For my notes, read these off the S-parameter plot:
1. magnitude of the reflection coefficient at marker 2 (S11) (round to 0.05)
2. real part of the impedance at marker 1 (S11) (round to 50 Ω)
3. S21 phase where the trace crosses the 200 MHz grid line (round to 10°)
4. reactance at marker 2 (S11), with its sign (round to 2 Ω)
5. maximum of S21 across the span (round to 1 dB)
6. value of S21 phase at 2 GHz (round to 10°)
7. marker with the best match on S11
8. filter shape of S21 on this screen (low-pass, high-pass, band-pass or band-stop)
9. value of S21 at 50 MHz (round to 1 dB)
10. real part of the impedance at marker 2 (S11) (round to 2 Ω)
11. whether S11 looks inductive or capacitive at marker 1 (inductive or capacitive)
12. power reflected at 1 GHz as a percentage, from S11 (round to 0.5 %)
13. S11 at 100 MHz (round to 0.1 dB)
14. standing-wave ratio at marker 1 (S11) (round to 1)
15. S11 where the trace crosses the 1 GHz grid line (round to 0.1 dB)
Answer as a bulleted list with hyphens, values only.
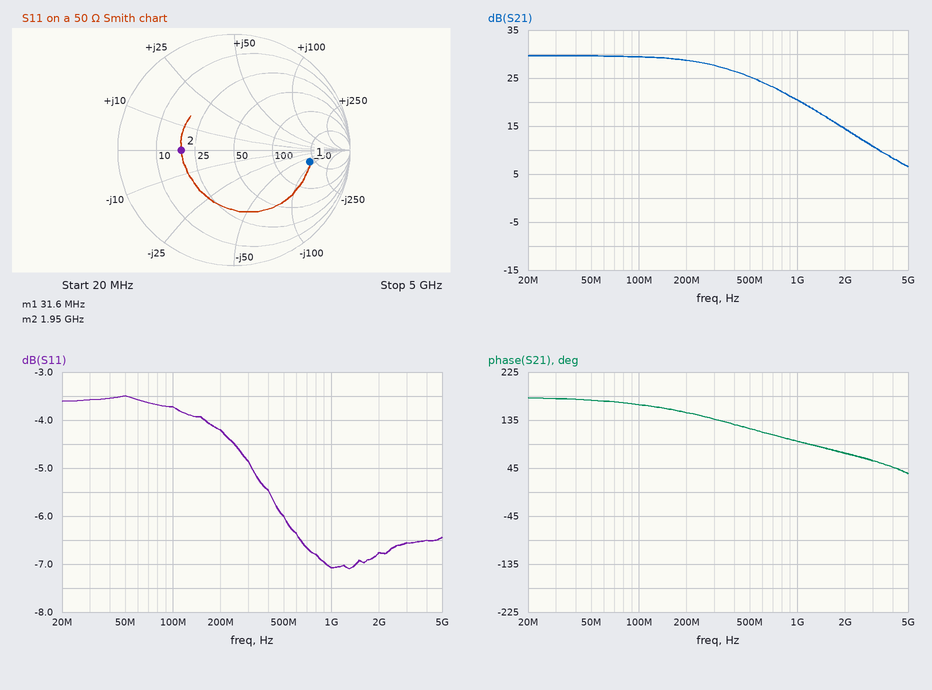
- 0.45
- 200 Ω
- 150°
- 0 Ω
- 30 dB
- 70°
- marker 2
- low-pass
- 30 dB
- 18 Ω
- capacitive
- 19.5 %
- -3.7 dB
- 5
- -7.1 dB
